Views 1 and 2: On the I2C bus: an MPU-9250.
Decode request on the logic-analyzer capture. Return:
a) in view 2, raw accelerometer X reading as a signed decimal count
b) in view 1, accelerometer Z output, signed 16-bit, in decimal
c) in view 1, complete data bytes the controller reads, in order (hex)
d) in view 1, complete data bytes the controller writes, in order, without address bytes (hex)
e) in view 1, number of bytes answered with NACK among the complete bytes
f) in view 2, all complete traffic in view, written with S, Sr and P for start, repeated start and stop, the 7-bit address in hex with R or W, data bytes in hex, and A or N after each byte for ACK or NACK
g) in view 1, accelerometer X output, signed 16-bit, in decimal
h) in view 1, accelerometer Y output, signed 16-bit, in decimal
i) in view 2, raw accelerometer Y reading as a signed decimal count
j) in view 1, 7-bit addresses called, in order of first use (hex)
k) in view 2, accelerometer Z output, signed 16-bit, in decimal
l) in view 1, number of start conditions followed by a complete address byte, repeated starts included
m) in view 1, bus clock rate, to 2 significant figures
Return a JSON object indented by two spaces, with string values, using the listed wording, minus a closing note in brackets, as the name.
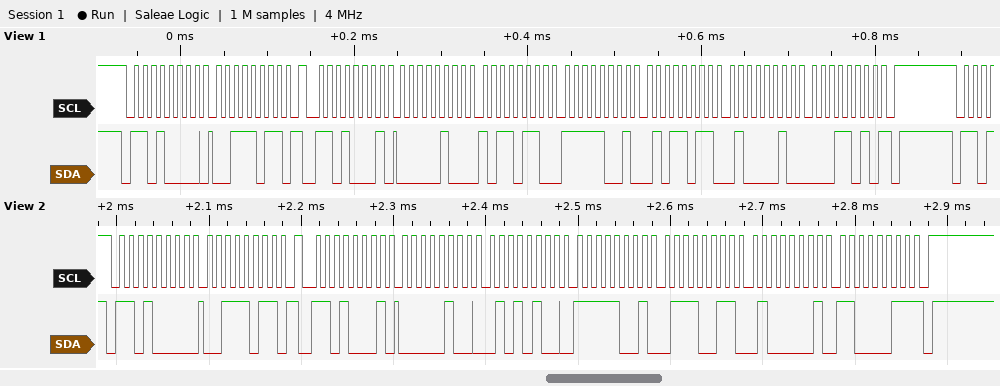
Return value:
{
  "in view 2, raw accelerometer X reading as a signed decimal count": "1108",
  "in view 1, accelerometer Z output, signed 16-bit, in decimal": "16922",
  "in view 1, complete data bytes the controller reads, in order": "04 B6 F9 5B 42 1A",
  "in view 1, complete data bytes the controller writes, in order, without address bytes": "3B",
  "in view 1, number of bytes answered with NACK among the complete bytes": "1",
  "in view 2, all complete traffic in view, written with S, Sr and P for start, repeated start and stop, the 7-bit address in hex with R or W, data bytes in hex, and A or N after each byte for ACK or NACK": "S 68W A 3B A Sr 68R A 04 A 54 A F9 A 73 A 41 A C3 N P",
  "in view 1, accelerometer X output, signed 16-bit, in decimal": "1206",
  "in view 1, accelerometer Y output, signed 16-bit, in decimal": "-1701",
  "in view 2, raw accelerometer Y reading as a signed decimal count": "-1677",
  "in view 1, 7-bit addresses called, in order of first use": "0x68",
  "in view 2, accelerometer Z output, signed 16-bit, in decimal": "16835",
  "in view 1, number of start conditions followed by a complete address byte, repeated starts included": "2",
  "in view 1, bus clock rate, to 2 significant figures": "100 kHz"
}
